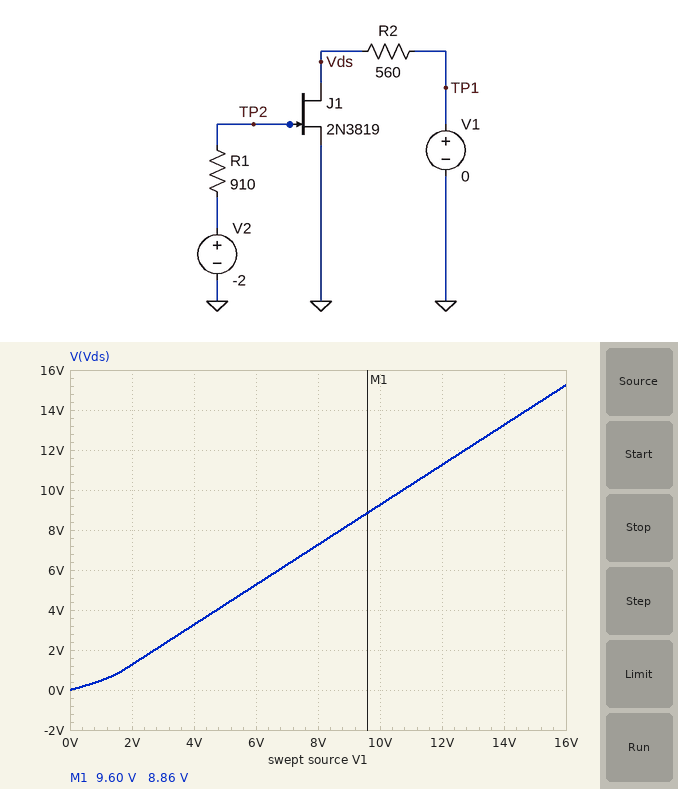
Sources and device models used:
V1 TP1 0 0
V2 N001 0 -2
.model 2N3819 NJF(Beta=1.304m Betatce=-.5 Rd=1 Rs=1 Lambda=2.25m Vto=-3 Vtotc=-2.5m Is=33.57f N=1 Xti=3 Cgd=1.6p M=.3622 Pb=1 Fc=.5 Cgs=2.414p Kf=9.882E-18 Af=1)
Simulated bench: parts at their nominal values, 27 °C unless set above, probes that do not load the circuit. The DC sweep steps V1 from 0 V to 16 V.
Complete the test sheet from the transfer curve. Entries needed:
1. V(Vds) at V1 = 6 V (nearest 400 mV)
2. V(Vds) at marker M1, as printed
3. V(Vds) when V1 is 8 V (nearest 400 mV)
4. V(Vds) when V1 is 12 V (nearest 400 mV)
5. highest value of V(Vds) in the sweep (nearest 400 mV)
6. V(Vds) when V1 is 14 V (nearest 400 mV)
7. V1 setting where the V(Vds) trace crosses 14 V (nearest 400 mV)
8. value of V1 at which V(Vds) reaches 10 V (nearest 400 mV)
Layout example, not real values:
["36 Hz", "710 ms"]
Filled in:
["5.2 V", "8.86 V", "7.2 V", "11.2 V", "15.2 V", "13.2 V", "14.8 V", "10.8 V"]
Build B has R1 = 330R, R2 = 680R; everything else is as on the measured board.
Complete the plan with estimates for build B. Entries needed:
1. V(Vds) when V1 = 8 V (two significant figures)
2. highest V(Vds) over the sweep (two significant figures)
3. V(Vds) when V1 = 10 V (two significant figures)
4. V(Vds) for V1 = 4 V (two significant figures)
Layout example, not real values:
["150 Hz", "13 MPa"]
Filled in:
["7.1 V", "15 V", "9.1 V", "3.1 V"]
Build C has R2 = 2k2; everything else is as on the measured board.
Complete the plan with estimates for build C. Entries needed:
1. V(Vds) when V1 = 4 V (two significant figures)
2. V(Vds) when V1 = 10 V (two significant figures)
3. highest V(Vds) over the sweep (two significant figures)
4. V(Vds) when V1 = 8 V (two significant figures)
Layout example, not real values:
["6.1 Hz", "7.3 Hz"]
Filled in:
["1.1 V", "7.1 V", "13 V", "5.1 V"]
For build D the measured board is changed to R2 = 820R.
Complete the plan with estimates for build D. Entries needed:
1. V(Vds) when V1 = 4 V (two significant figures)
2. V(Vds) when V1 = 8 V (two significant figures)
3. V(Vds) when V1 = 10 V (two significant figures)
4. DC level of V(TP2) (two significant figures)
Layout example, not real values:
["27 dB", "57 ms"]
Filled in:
["2.9 V", "6.9 V", "8.9 V", "-2.0 V"]
